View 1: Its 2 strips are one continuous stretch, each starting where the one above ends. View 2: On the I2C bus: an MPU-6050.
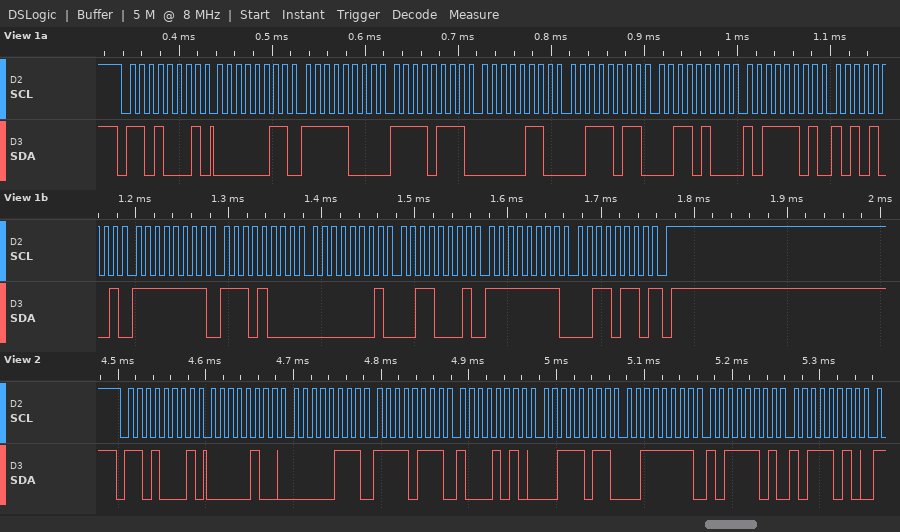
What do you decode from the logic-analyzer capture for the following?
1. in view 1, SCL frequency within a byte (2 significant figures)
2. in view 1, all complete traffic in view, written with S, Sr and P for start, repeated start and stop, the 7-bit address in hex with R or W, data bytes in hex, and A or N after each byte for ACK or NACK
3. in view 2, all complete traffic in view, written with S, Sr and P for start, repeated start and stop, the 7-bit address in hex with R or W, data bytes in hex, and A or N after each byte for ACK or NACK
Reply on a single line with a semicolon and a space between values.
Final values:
100 kHz; S 68R A 03 A F8 A F7 A 06 A 3B A 34 A BD A A9 A FF A E8 A 01 A 31 A FF A 36 N P; S 68R A 04 A 07 A F7 A 8A A 3B A 3F A BD A BA A
